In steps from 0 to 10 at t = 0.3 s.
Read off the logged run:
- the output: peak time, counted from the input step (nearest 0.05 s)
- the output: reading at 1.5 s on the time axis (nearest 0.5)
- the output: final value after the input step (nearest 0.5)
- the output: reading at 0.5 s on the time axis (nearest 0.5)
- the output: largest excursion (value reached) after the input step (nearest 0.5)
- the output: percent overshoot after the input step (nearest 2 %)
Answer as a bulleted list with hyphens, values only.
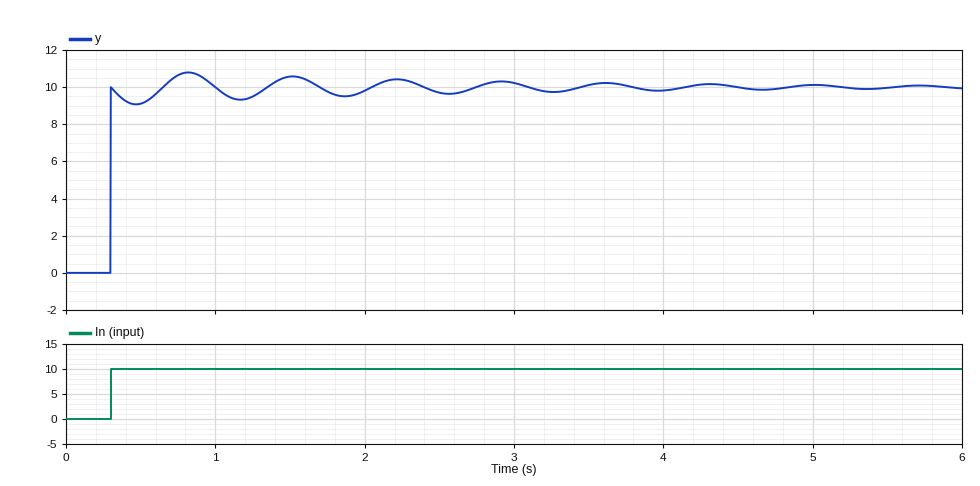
- 0.50 s
- 10.5
- 10.0
- 9.0
- 11.0
- 8 %
